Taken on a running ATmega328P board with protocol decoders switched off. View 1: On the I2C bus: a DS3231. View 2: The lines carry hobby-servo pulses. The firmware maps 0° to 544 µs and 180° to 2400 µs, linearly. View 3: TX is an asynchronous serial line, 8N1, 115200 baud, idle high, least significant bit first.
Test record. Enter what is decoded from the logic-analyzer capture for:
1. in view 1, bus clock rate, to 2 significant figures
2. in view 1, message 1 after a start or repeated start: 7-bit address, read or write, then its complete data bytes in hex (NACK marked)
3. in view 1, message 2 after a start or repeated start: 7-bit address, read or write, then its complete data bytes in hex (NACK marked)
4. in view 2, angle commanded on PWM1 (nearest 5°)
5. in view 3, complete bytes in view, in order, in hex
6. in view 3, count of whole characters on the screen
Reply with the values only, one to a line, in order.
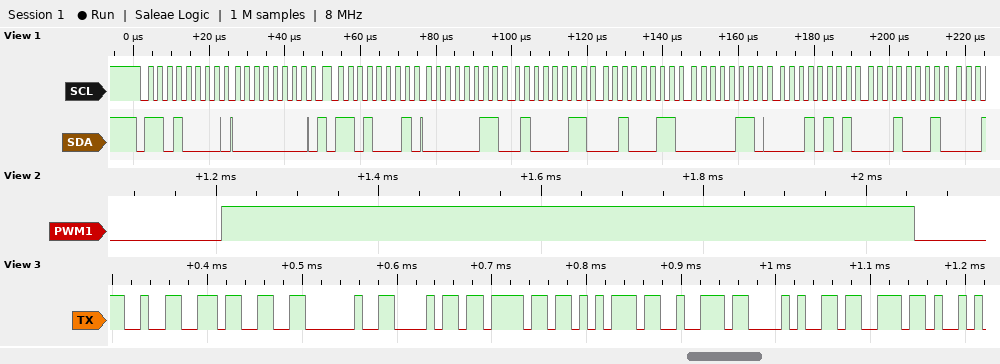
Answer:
400 kHz
0x68 write: 00
0x68 read: 03 43 23 06 15 11
30°
32 33 20 68 6F 75 72 28 73
9
